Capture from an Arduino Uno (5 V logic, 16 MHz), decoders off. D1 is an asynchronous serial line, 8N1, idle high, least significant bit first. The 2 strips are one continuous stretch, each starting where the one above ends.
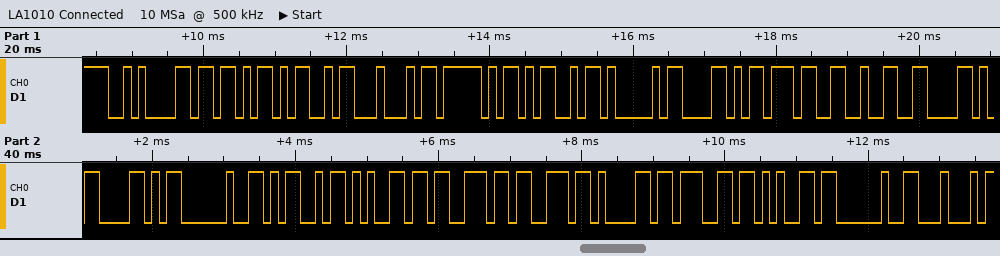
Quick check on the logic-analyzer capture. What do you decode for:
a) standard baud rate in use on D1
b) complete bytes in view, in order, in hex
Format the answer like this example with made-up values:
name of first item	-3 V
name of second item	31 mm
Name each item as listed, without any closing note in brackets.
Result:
standard baud rate in use on D1	9600 baud
complete bytes in view, in order, in hex	0x0A 0x5B 0x4D 0x44 0x5F 0x4D 0x41 0x58 0x37 0x32 0x58 0x58 0x20 0x4D 0x65 0x73 0x73 0x61 0x67 0x65 0x20 0x44
